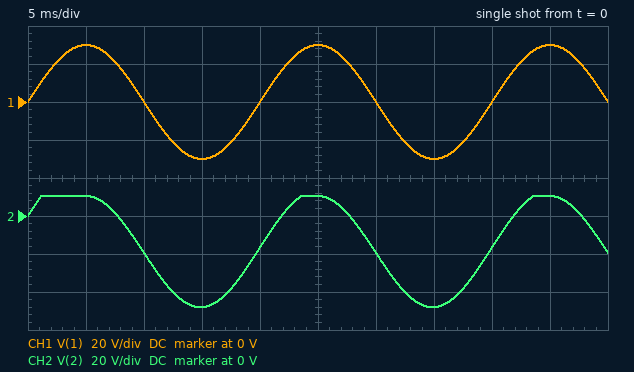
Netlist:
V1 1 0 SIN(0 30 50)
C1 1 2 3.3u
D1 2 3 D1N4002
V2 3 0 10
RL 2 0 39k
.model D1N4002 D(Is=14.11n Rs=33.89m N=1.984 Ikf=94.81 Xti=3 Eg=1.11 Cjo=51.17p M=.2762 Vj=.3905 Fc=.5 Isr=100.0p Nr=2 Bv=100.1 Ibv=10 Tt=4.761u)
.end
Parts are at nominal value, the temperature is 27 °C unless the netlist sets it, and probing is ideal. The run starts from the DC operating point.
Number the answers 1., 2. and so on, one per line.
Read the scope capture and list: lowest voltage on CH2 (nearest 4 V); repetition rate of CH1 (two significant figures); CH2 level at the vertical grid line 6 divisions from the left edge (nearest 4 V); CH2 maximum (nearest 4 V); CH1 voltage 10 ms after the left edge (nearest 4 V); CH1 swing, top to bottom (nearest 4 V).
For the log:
1. -48 V
2. 50 Hz
3. -20 V
4. 12 V
5. 0 V
6. 60 V
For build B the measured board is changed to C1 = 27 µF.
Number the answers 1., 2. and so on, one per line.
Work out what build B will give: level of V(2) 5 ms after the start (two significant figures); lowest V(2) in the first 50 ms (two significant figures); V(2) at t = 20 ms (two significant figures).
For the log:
1. 11 V
2. -49 V
3. -19 V
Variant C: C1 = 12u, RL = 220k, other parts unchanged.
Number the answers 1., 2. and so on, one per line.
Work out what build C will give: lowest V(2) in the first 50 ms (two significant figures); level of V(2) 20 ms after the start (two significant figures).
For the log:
1. -49 V
2. -19 V
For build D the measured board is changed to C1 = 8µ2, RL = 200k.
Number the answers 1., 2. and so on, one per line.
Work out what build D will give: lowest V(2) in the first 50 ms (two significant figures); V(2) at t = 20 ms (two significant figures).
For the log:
1. -49 V
2. -19 V
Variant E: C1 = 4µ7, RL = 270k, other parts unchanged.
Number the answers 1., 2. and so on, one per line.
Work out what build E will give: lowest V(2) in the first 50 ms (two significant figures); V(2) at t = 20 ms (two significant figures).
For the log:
1. -49 V
2. -19 V
